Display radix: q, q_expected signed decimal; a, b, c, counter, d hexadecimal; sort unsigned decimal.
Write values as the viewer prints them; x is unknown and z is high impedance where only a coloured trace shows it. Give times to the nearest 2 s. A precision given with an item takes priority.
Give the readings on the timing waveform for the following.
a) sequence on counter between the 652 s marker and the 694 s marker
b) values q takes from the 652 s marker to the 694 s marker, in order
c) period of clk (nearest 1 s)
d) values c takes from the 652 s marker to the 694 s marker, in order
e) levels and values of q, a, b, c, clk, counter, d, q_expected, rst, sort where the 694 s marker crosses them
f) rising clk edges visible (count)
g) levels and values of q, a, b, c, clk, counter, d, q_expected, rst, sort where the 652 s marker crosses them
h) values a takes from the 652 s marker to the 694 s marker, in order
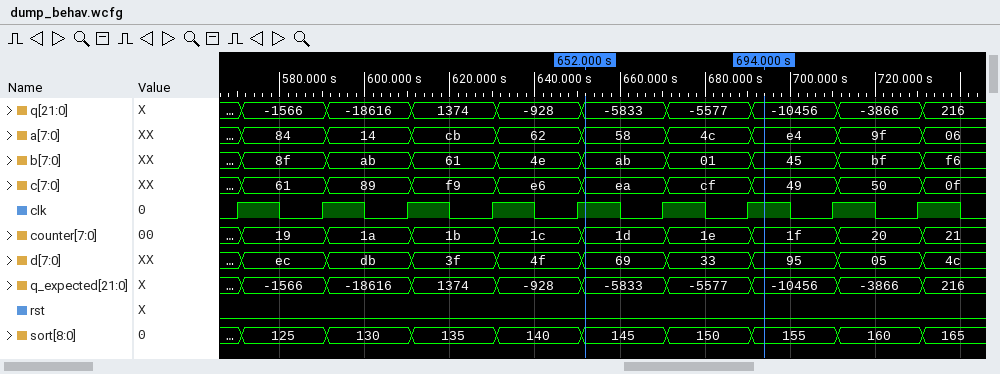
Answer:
1d, 1e, 1f
-5833, -5577, -10456
20 s
ea, cf, 49
q=-10456, a=e4, b=45, c=49, clk=1, counter=1f, d=95, q_expected=-10456, rst=0, sort=155
9
q=-5833, a=58, b=ab, c=ea, clk=1, counter=1d, d=69, q_expected=-5833, rst=0, sort=145
58, 4c, e4
